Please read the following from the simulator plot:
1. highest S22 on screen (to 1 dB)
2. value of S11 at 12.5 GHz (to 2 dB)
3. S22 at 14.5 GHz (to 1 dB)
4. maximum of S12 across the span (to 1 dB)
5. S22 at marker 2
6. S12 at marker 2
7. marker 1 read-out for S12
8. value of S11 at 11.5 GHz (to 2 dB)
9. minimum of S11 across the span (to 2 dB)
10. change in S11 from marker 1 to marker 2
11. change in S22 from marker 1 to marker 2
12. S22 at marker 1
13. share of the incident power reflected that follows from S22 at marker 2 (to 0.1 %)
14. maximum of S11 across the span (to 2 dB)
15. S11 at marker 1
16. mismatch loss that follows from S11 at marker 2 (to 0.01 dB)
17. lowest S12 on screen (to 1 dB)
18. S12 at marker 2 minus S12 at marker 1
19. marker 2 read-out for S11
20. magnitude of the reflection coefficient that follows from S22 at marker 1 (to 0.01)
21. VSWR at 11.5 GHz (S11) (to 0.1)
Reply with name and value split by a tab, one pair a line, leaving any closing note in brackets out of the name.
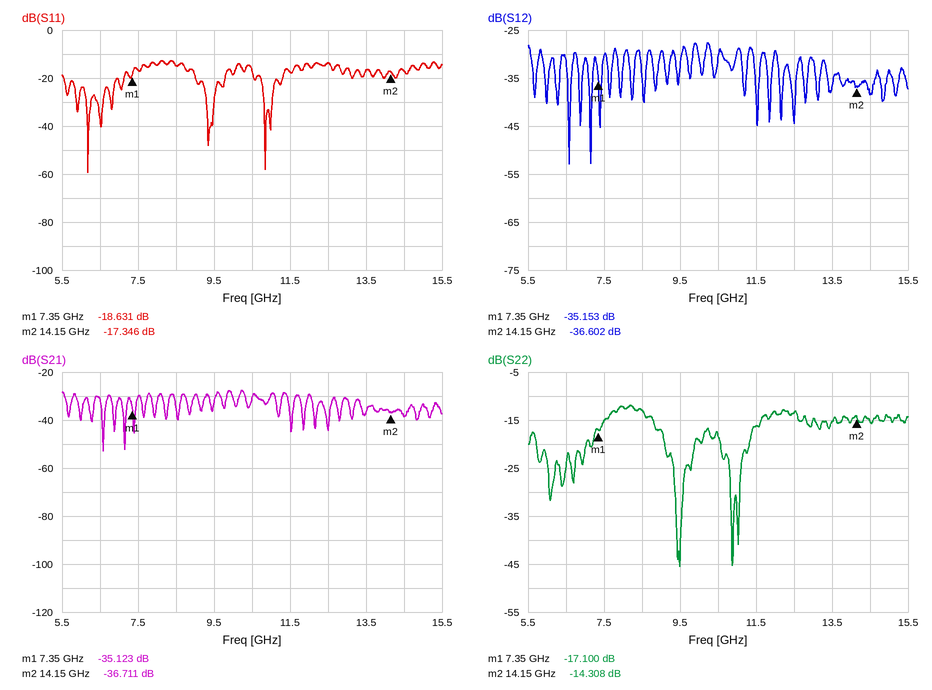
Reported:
highest S22 on screen	-12 dB
value of S11 at 12.5 GHz	-14 dB
S22 at 14.5 GHz	-15 dB
maximum of S12 across the span	-28 dB
S22 at marker 2	-14.308 dB
S12 at marker 2	-36.602 dB
marker 1 read-out for S12	-35.153 dB
value of S11 at 11.5 GHz	-18 dB
minimum of S11 across the span	-60 dB
change in S11 from marker 1 to marker 2	1.285 dB
change in S22 from marker 1 to marker 2	2.792 dB
S22 at marker 1	-17.100 dB
share of the incident power reflected that follows from S22 at marker 2	3.7 %
maximum of S11 across the span	-12 dB
S11 at marker 1	-18.631 dB
mismatch loss that follows from S11 at marker 2	0.08 dB
lowest S12 on screen	-53 dB
S12 at marker 2 minus S12 at marker 1	-1.449 dB
marker 2 read-out for S11	-17.346 dB
magnitude of the reflection coefficient that follows from S22 at marker 1	0.14
VSWR at 11.5 GHz (S11)	1.3
